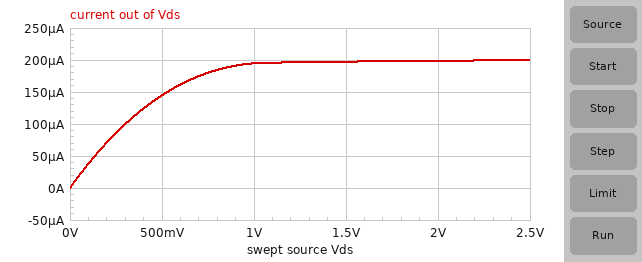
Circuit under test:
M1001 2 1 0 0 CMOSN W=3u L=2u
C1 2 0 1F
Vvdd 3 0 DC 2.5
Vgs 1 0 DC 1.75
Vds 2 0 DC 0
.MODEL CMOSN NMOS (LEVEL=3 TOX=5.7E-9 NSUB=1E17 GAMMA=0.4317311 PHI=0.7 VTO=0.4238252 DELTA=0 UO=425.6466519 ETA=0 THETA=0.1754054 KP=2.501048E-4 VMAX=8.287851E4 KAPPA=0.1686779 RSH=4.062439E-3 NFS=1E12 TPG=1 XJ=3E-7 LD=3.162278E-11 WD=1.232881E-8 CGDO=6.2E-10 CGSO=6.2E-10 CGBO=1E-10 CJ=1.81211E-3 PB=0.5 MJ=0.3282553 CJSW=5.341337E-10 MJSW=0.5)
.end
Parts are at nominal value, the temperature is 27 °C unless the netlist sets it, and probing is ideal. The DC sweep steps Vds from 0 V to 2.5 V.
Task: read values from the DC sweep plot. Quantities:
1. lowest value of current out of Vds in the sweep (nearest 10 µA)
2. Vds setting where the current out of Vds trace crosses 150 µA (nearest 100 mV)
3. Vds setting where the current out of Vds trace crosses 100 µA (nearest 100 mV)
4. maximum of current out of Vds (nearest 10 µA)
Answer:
0 A
500 mV
300 mV
200 µA
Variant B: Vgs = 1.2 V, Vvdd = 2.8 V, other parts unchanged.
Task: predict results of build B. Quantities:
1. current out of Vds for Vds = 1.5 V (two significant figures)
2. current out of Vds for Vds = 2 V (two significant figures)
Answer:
80 µA
81 µA
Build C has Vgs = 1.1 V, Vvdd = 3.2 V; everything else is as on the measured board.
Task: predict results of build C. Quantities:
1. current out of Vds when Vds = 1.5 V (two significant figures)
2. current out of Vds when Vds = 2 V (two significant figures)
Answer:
63 µA
64 µA
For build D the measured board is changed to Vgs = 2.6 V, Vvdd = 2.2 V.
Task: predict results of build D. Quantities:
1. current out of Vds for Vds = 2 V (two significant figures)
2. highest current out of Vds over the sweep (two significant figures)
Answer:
430 µA
440 µA
